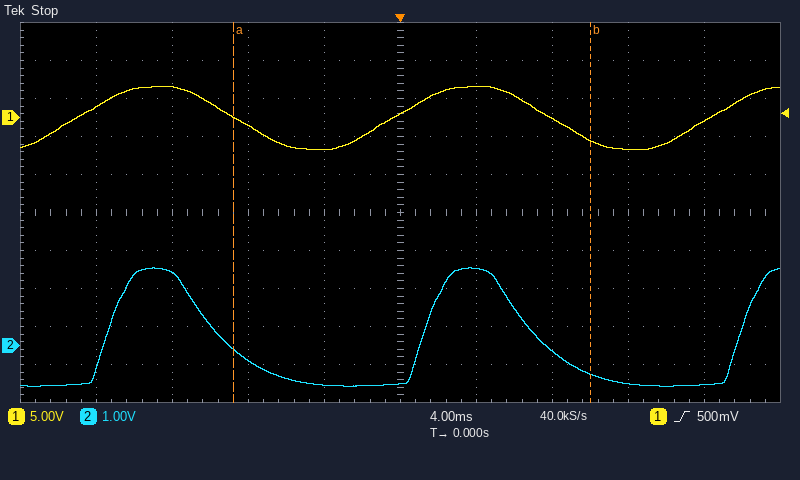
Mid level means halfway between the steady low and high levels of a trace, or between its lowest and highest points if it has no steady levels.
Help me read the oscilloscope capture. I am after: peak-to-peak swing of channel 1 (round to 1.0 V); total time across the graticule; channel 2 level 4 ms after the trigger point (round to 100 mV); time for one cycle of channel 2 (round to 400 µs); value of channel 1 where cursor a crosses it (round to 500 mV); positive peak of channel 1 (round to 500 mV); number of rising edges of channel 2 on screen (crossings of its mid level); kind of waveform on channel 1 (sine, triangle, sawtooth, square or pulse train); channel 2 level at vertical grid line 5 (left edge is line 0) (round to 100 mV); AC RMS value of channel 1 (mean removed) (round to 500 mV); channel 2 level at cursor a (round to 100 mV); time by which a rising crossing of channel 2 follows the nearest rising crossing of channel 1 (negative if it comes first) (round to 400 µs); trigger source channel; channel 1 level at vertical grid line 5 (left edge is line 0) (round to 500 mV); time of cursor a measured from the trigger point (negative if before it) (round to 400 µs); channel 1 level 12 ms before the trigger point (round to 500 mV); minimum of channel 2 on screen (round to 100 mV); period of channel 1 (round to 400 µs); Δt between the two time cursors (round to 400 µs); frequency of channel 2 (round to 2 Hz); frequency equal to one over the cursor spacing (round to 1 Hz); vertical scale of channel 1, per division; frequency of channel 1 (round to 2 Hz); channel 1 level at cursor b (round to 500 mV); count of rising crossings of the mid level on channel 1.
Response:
8.0 V
40 ms
2.0 V
16.8 ms
0.0 V
4.0 V
3
sine
-1.0 V
3.0 V
-100 mV
+1.6 ms
channel 1
500 mV
-8.8 ms
4.0 V
-1.1 V
16.8 ms
18.8 ms
60 Hz
53 Hz
5 V
60 Hz
-3.0 V
3
